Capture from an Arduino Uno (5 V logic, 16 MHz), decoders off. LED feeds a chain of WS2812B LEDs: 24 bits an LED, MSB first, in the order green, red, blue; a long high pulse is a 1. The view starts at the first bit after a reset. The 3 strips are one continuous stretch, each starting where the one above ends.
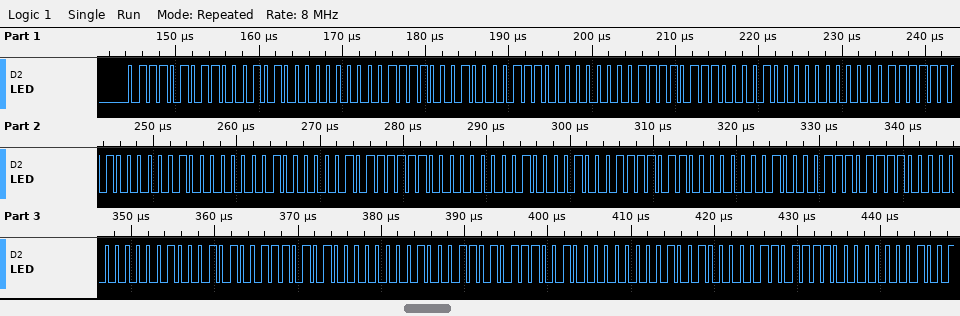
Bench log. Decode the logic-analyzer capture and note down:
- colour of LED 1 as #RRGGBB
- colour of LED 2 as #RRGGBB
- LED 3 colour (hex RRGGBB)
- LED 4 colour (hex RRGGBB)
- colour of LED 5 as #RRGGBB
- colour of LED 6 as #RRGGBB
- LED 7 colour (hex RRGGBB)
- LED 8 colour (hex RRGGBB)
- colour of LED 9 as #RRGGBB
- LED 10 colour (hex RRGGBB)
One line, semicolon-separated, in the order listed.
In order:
#8A7500; #877800; #847B00; #817E00; #7E8100; #7B8400; #788700; #758A00; #728D00; #6F9000
